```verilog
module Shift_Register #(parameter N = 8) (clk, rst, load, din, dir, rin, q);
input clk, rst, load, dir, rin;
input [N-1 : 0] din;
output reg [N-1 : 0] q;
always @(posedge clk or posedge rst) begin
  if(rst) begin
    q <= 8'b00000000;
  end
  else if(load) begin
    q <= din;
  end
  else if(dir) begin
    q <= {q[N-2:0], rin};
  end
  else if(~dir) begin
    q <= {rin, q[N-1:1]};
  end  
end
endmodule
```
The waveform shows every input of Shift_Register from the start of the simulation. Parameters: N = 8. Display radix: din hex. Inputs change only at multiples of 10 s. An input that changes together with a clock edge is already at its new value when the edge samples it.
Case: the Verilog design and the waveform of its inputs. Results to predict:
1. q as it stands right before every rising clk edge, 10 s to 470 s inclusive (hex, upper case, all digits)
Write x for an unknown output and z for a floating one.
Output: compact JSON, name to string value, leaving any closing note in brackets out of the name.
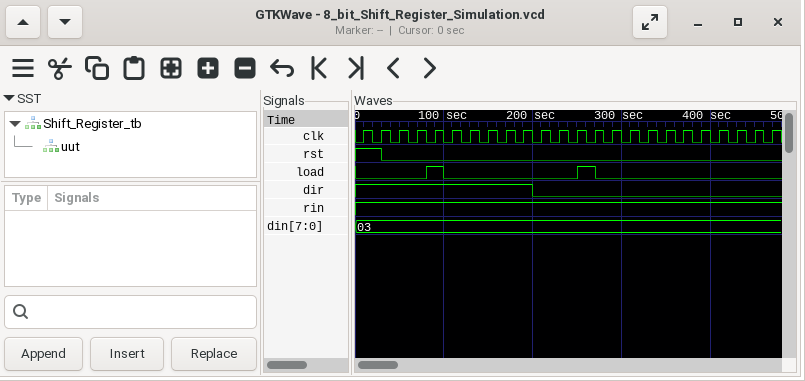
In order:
{"q as it stands right before every rising clk edge, 10 s to 470 s inclusive": "00, 00, 01, 03, 07, 03, 07, 0F, 1F, 3F, 7F, BF, DF, 03, 81, C0, E0, F0, F8, FC, FE, FF, FF, FF"}
